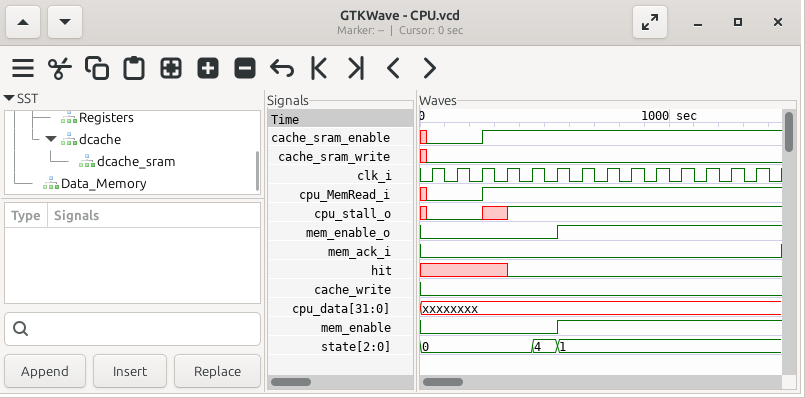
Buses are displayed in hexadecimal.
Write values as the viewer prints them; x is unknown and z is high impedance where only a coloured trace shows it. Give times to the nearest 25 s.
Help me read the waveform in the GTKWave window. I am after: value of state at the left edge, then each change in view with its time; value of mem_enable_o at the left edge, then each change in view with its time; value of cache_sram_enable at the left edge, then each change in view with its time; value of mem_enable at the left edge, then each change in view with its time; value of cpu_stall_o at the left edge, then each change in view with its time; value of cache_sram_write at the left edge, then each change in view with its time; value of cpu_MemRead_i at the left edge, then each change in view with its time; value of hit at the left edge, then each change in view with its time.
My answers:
0, 4 at 450 s, 1 at 550 s
0, 1 at 550 s
x, 0 at 25 s, 1 at 250 s
0, 1 at 550 s
x, 0 at 25 s, x at 250 s, 1 at 350 s
x, 0 at 25 s
x, 0 at 25 s, 1 at 250 s
x, 0 at 350 s
